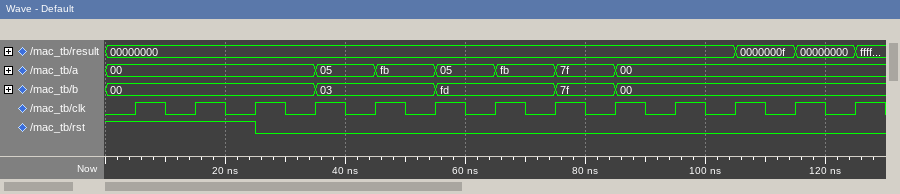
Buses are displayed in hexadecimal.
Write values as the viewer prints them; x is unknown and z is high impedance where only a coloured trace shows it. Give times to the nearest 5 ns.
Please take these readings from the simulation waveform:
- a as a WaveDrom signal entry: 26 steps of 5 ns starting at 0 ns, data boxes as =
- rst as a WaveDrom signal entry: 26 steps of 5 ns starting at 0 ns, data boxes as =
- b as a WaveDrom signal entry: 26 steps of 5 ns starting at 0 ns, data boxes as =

{name: 'a', wave: '=......=.=.=.=.=.=........', data: '00 05 fb 05 fb 7f 00'}
{name: 'rst', wave: '1....0....................'}
{name: 'b', wave: '=......=...=...=.=........', data: '00 03 fd 7f 00'}
